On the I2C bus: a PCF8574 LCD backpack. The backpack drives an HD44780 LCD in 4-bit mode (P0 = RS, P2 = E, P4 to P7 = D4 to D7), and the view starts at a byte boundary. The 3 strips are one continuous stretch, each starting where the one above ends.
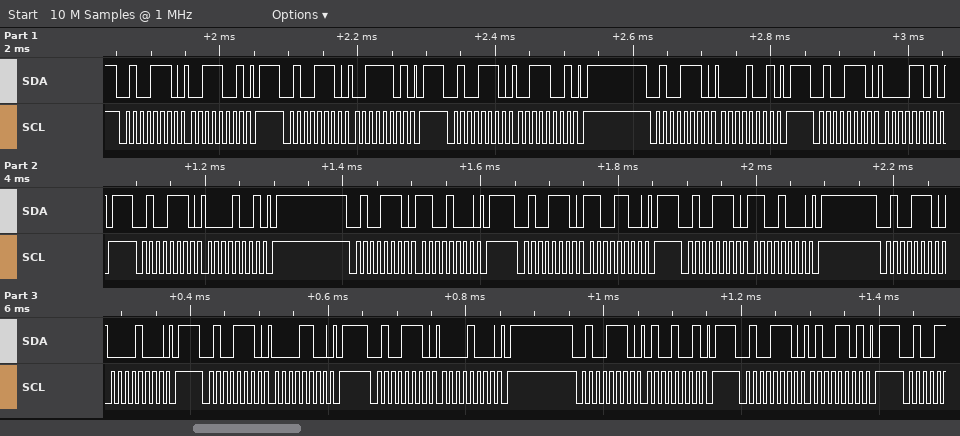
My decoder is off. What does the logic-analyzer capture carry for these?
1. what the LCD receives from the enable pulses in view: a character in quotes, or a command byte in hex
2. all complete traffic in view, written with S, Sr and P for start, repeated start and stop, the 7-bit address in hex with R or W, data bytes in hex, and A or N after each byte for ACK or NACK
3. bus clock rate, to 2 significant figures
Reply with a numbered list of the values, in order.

1. '0' 0xC0
2. S 27W A 39 A P S 27W A 3D A P S 27W A 39 A P S 27W A 09 A P S 27W A 0D A P S 27W A 09 A P S 27W A C8 A P S 27W A CC A P S 27W A C8 A P S 27W A 08 A P S 27W A 0C A P S 27W A 08 A P S 27W A 49 A P S 27W A 4D A P
3. 100 kHz
